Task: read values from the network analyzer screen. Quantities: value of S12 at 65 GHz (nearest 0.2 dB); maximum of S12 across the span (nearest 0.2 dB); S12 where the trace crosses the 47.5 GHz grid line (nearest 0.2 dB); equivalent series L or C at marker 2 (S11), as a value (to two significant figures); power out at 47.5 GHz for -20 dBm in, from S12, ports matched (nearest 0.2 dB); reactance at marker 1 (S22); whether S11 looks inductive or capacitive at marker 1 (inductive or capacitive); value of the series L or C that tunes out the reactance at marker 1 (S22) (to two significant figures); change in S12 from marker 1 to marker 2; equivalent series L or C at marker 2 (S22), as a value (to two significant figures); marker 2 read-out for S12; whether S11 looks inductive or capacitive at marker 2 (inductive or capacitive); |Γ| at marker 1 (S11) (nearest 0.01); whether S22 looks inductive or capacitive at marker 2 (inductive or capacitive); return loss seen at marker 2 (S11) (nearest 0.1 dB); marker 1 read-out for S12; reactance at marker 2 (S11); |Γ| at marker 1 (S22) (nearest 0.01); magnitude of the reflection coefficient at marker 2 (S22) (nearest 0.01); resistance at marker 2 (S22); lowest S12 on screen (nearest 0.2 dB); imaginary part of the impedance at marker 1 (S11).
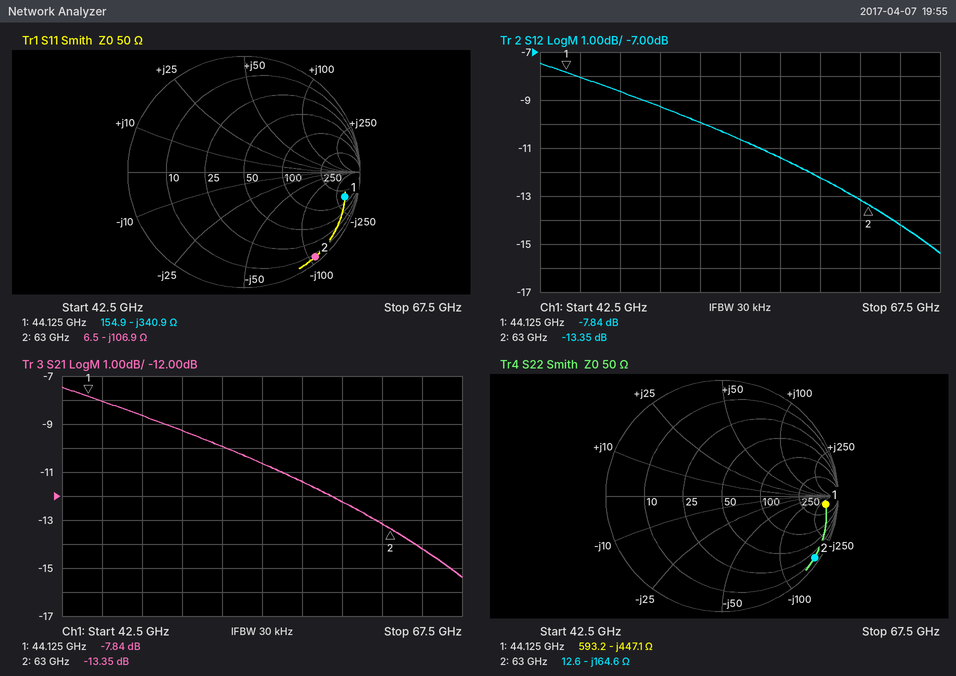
-14.2 dB
-7.4 dB
-8.6 dB
24 fF
-28.6 dBm
-447.1 Ω
capacitive
1.6 nH
-5.51 dB
15 fF
-13.35 dB
capacitive
0.90
capacitive
0.4 dB
-7.84 dB
-106.9 Ω
0.90
0.96
12.6 Ω
-15.4 dB
-340.9 Ω
